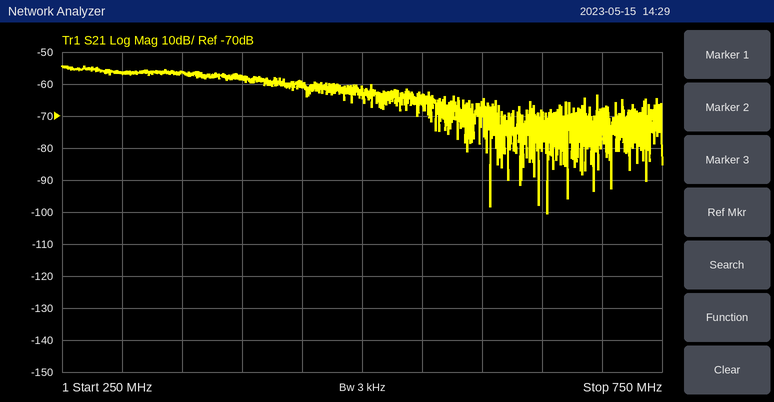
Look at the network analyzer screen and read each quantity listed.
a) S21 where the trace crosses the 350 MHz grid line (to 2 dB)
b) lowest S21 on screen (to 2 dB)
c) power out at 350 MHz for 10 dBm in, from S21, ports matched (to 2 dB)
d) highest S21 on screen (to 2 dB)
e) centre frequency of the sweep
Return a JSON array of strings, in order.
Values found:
["-56 dB", "-100 dB", "-46 dBm", "-54 dB", "500 MHz"]
